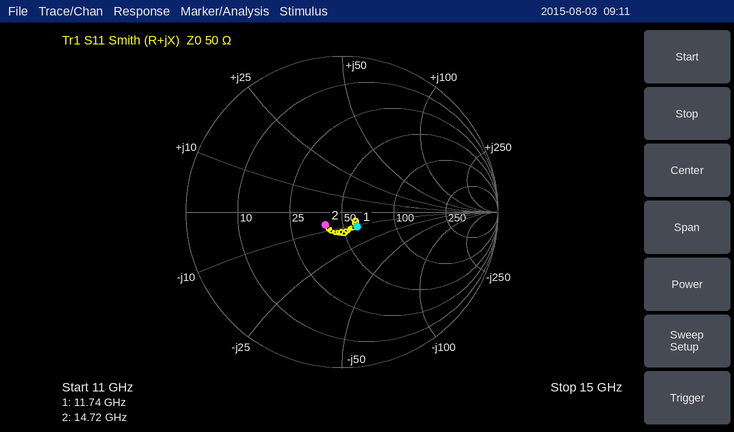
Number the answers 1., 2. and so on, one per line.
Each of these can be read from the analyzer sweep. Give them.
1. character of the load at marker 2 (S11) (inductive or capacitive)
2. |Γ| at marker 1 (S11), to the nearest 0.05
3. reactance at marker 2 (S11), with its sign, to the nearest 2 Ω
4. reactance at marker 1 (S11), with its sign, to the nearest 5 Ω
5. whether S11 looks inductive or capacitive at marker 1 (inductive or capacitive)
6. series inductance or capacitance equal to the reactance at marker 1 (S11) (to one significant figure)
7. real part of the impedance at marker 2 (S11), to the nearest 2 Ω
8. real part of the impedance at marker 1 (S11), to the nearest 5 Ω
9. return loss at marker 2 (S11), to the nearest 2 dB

1. capacitive
2. 0.15
3. -6 Ω
4. -10 Ω
5. capacitive
6. 1 pF
7. 40 Ω
8. 60 Ω
9. 18 dB
